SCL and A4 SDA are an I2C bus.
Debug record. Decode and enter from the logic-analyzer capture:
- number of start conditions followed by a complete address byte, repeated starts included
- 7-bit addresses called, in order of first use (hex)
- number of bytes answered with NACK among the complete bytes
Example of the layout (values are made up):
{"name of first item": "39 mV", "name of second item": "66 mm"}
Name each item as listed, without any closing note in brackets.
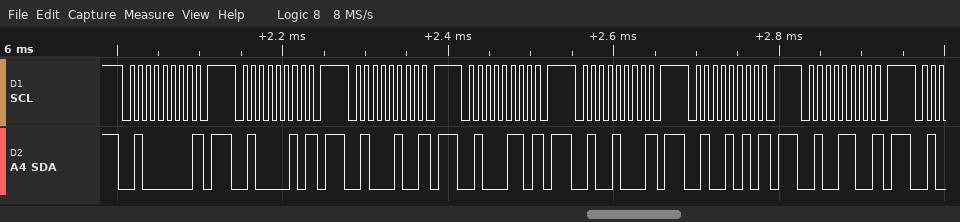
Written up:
{"number of start conditions followed by a complete address byte, repeated starts included": "7", "7-bit addresses called, in order of first use": "0x20 0x21 0x22 0x23 0x24 0x25 0x26", "number of bytes answered with NACK among the complete bytes": "7"}
